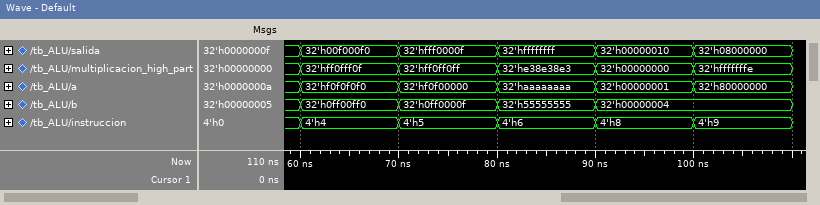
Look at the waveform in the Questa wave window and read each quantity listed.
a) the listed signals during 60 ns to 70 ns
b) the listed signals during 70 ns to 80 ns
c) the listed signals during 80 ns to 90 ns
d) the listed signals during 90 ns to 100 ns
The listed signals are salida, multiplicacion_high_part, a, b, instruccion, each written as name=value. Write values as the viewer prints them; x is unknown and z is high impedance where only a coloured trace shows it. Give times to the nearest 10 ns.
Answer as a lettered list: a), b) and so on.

a) salida=32'h00f000f0, multiplicacion_high_part=32'hff0fff0f, a=32'hf0f0f0f0, b=32'h0ff00ff0, instruccion=4'h4
b) salida=32'hfff0000f, multiplicacion_high_part=32'hff0ff0ff, a=32'hf0f00000, b=32'h0ff0000f, instruccion=4'h5
c) salida=32'hffffffff, multiplicacion_high_part=32'he38e38e3, a=32'haaaaaaaa, b=32'h55555555, instruccion=4'h6
d) salida=32'h00000010, multiplicacion_high_part=32'h00000000, a=32'h00000001, b=32'h00000004, instruccion=4'h8
